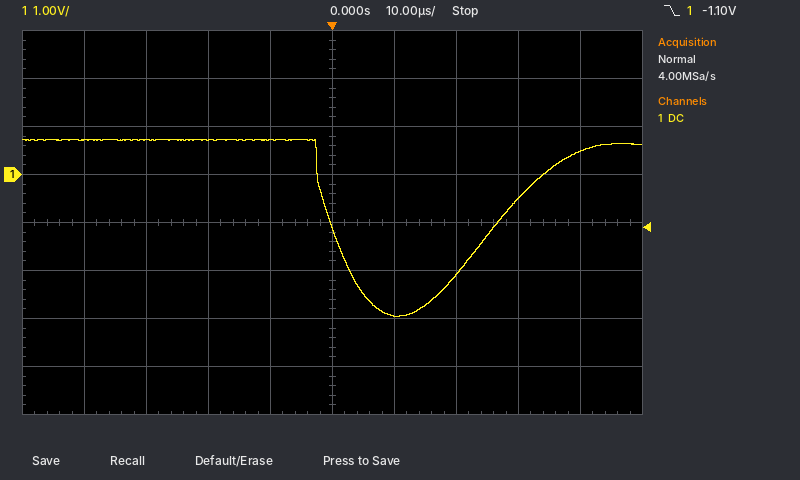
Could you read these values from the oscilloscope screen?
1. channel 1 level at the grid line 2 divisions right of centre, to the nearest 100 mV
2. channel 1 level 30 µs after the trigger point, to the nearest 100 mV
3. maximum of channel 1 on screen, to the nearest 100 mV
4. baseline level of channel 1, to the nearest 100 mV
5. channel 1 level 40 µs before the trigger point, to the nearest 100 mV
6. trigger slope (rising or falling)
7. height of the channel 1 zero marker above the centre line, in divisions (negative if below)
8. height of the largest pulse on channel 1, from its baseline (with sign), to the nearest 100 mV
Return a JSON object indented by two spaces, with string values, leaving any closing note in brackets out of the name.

{
  "channel 1 level at the grid line 2 divisions right of centre, to the nearest 100 mV": "-2.1 V",
  "channel 1 level 30 µs after the trigger point, to the nearest 100 mV": "-500 mV",
  "maximum of channel 1 on screen, to the nearest 100 mV": "700 mV",
  "baseline level of channel 1, to the nearest 100 mV": "700 mV",
  "channel 1 level 40 µs before the trigger point, to the nearest 100 mV": "700 mV",
  "trigger slope": "falling",
  "height of the channel 1 zero marker above the centre line, in divisions": "+1.0 div",
  "height of the largest pulse on channel 1, from its baseline (with sign), to the nearest 100 mV": "-3.7 V"
}
